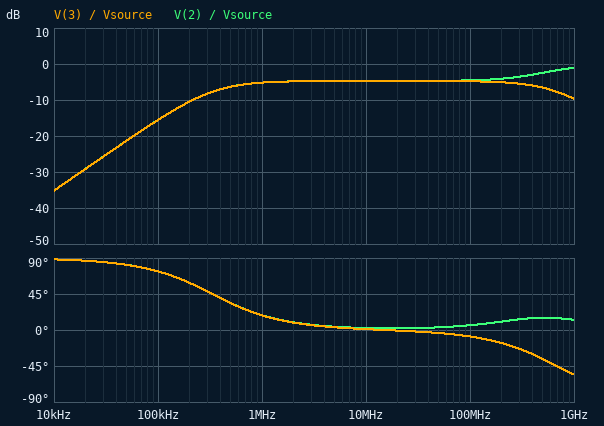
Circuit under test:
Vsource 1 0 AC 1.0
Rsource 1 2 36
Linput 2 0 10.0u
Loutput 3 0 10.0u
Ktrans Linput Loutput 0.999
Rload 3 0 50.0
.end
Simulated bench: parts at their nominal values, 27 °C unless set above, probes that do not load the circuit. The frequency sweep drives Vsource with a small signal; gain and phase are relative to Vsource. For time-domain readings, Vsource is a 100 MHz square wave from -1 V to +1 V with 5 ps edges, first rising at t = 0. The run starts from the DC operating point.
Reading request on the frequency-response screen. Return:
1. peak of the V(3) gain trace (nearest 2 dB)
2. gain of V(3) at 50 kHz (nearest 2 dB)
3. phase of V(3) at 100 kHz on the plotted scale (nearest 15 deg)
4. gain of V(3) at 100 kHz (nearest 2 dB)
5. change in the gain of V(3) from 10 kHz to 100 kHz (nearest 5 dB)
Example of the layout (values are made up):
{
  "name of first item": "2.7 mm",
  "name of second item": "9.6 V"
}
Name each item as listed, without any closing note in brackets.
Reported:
{
  "peak of the V(3) gain trace": "-4 dB",
  "gain of V(3) at 50 kHz": "-22 dB",
  "phase of V(3) at 100 kHz on the plotted scale": "75 deg",
  "gain of V(3) at 100 kHz": "-16 dB",
  "change in the gain of V(3) from 10 kHz to 100 kHz": "20 dB"
}
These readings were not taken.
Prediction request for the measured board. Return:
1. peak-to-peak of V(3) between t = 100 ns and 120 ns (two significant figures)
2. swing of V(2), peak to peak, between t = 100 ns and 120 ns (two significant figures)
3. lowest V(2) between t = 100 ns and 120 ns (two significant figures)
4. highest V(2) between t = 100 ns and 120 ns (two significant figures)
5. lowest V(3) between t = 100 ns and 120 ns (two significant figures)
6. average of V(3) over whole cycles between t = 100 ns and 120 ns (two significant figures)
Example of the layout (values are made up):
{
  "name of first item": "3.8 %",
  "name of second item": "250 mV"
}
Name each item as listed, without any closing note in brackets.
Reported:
{
  "peak-to-peak of V(3) between t = 100 ns and 120 ns": "1.2 V",
  "swing of V(2), peak to peak, between t = 100 ns and 120 ns": "2.8 V",
  "lowest V(2) between t = 100 ns and 120 ns": "-960 mV",
  "highest V(2) between t = 100 ns and 120 ns": "1.9 V",
  "lowest V(3) between t = 100 ns and 120 ns": "-130 mV",
  "average of V(3) over whole cycles between t = 100 ns and 120 ns": "460 mV"
}
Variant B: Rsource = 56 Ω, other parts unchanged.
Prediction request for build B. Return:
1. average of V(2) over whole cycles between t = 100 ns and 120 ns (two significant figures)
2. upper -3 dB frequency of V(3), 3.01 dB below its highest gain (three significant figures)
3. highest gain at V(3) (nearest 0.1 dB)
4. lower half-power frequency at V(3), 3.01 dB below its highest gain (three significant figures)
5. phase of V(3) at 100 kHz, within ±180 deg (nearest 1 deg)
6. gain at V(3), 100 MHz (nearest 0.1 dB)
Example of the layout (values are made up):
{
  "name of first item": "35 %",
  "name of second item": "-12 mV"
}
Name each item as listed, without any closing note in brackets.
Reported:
{
  "average of V(2) over whole cycles between t = 100 ns and 120 ns": "350 mV",
  "upper -3 dB frequency of V(3), 3.01 dB below its highest gain": "844 MHz",
  "highest gain at V(3)": "-6.5 dB",
  "lower half-power frequency at V(3), 3.01 dB below its highest gain": "420 kHz",
  "phase of V(3) at 100 kHz, within ±180 deg": "77 deg",
  "gain at V(3), 100 MHz": "-6.6 dB"
}
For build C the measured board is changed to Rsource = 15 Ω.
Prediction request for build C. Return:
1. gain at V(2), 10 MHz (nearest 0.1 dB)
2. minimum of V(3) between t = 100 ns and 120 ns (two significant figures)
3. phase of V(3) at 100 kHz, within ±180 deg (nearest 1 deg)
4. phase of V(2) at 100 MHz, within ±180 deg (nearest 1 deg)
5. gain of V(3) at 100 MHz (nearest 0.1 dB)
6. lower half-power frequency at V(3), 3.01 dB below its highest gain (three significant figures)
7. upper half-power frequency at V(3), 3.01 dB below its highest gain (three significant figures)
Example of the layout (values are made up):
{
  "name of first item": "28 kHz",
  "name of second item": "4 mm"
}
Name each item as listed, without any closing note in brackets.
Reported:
{
  "gain at V(2), 10 MHz": "-2.3 dB",
  "minimum of V(3) between t = 100 ns and 120 ns": "-99 mV",
  "phase of V(3) at 100 kHz, within ±180 deg": "61 deg",
  "phase of V(2) at 100 MHz, within ±180 deg": "3 deg",
  "gain of V(3) at 100 MHz": "-2.4 dB",
  "lower half-power frequency at V(3), 3.01 dB below its highest gain": "184 kHz",
  "upper half-power frequency at V(3), 3.01 dB below its highest gain": "518 MHz"
}
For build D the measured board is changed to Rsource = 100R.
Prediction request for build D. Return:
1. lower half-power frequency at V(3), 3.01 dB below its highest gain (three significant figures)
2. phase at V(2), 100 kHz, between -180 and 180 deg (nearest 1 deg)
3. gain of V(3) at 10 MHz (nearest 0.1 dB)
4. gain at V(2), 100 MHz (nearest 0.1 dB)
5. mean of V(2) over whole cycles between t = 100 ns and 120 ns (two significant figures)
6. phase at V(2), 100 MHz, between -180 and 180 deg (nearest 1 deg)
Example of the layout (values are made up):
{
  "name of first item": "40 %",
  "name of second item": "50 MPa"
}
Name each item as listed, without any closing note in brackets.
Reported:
{
  "lower half-power frequency at V(3), 3.01 dB below its highest gain": "530 kHz",
  "phase at V(2), 100 kHz, between -180 and 180 deg": "79 deg",
  "gain of V(3) at 10 MHz": "-9.6 dB",
  "gain at V(2), 100 MHz": "-9.3 dB",
  "mean of V(2) over whole cycles between t = 100 ns and 120 ns": "230 mV",
  "phase at V(2), 100 MHz, between -180 and 180 deg": "10 deg"
}
